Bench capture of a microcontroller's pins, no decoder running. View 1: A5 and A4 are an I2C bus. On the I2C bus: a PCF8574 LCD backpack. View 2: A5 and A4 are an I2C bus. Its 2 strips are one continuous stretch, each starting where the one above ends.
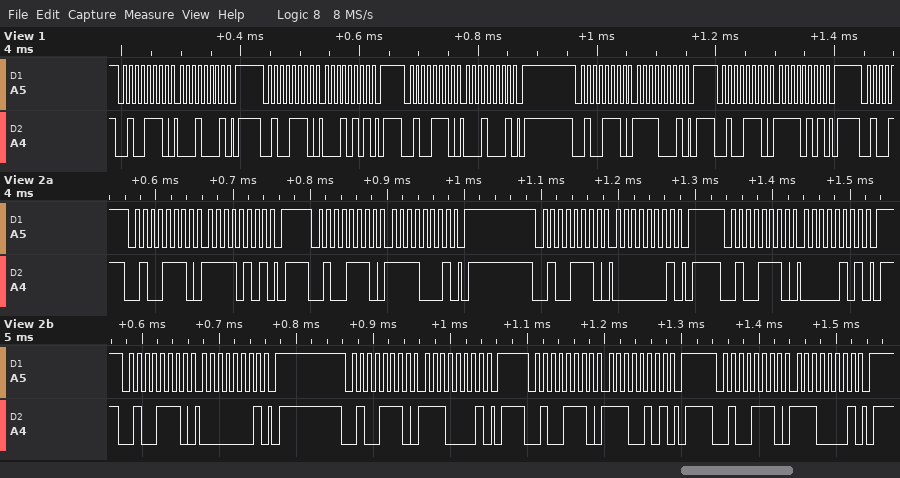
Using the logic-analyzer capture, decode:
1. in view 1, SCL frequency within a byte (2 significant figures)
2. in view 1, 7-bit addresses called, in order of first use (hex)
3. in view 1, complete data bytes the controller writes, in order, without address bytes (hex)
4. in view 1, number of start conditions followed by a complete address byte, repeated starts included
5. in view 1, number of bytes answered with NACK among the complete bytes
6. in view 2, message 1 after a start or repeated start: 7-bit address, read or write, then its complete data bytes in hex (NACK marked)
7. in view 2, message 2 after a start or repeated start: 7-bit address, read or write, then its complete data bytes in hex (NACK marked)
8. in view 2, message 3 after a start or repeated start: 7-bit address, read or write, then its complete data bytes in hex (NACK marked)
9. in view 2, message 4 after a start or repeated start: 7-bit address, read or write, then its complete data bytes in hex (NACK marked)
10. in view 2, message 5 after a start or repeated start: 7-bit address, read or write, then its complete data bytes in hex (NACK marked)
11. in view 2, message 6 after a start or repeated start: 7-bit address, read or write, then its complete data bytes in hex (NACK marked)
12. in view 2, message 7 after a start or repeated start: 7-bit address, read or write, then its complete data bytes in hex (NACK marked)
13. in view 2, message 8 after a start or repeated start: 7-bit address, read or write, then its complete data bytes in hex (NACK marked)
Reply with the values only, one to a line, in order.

100 kHz
0x27
11 15 11 F1 F5
5
0
0x27 write: F5
0x27 write: F1
0x27 write: 01
0x27 write: 05
0x27 write: 01
0x27 write: E1
0x27 write: E5
0x27 write: E1
